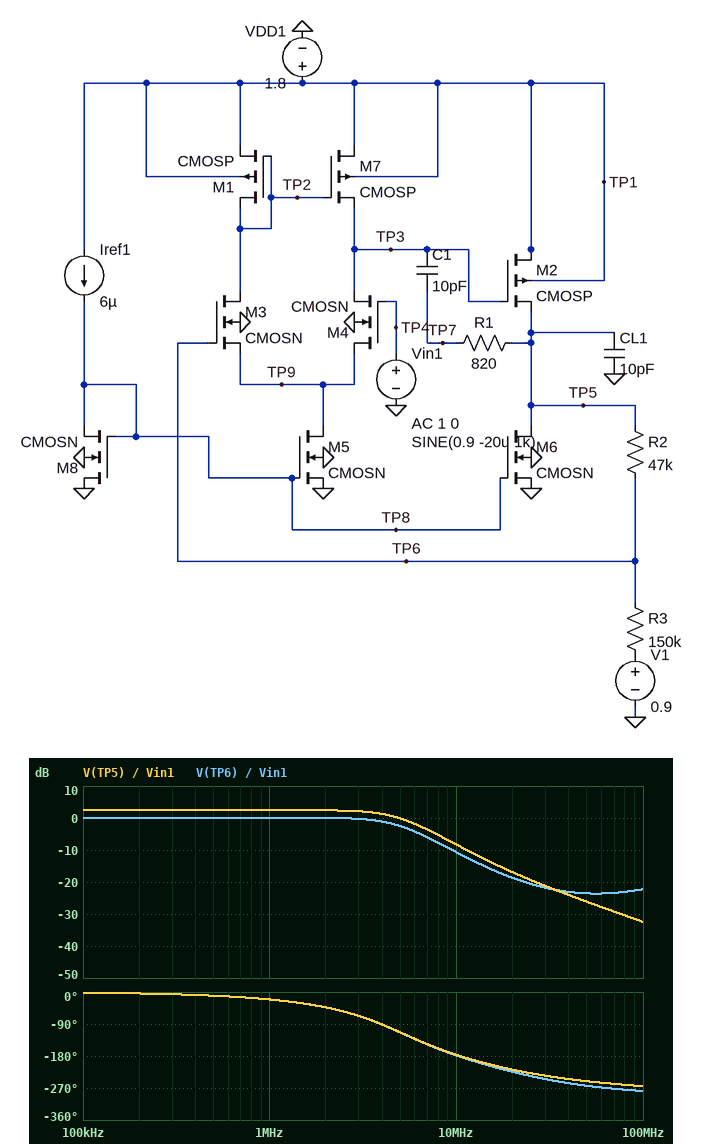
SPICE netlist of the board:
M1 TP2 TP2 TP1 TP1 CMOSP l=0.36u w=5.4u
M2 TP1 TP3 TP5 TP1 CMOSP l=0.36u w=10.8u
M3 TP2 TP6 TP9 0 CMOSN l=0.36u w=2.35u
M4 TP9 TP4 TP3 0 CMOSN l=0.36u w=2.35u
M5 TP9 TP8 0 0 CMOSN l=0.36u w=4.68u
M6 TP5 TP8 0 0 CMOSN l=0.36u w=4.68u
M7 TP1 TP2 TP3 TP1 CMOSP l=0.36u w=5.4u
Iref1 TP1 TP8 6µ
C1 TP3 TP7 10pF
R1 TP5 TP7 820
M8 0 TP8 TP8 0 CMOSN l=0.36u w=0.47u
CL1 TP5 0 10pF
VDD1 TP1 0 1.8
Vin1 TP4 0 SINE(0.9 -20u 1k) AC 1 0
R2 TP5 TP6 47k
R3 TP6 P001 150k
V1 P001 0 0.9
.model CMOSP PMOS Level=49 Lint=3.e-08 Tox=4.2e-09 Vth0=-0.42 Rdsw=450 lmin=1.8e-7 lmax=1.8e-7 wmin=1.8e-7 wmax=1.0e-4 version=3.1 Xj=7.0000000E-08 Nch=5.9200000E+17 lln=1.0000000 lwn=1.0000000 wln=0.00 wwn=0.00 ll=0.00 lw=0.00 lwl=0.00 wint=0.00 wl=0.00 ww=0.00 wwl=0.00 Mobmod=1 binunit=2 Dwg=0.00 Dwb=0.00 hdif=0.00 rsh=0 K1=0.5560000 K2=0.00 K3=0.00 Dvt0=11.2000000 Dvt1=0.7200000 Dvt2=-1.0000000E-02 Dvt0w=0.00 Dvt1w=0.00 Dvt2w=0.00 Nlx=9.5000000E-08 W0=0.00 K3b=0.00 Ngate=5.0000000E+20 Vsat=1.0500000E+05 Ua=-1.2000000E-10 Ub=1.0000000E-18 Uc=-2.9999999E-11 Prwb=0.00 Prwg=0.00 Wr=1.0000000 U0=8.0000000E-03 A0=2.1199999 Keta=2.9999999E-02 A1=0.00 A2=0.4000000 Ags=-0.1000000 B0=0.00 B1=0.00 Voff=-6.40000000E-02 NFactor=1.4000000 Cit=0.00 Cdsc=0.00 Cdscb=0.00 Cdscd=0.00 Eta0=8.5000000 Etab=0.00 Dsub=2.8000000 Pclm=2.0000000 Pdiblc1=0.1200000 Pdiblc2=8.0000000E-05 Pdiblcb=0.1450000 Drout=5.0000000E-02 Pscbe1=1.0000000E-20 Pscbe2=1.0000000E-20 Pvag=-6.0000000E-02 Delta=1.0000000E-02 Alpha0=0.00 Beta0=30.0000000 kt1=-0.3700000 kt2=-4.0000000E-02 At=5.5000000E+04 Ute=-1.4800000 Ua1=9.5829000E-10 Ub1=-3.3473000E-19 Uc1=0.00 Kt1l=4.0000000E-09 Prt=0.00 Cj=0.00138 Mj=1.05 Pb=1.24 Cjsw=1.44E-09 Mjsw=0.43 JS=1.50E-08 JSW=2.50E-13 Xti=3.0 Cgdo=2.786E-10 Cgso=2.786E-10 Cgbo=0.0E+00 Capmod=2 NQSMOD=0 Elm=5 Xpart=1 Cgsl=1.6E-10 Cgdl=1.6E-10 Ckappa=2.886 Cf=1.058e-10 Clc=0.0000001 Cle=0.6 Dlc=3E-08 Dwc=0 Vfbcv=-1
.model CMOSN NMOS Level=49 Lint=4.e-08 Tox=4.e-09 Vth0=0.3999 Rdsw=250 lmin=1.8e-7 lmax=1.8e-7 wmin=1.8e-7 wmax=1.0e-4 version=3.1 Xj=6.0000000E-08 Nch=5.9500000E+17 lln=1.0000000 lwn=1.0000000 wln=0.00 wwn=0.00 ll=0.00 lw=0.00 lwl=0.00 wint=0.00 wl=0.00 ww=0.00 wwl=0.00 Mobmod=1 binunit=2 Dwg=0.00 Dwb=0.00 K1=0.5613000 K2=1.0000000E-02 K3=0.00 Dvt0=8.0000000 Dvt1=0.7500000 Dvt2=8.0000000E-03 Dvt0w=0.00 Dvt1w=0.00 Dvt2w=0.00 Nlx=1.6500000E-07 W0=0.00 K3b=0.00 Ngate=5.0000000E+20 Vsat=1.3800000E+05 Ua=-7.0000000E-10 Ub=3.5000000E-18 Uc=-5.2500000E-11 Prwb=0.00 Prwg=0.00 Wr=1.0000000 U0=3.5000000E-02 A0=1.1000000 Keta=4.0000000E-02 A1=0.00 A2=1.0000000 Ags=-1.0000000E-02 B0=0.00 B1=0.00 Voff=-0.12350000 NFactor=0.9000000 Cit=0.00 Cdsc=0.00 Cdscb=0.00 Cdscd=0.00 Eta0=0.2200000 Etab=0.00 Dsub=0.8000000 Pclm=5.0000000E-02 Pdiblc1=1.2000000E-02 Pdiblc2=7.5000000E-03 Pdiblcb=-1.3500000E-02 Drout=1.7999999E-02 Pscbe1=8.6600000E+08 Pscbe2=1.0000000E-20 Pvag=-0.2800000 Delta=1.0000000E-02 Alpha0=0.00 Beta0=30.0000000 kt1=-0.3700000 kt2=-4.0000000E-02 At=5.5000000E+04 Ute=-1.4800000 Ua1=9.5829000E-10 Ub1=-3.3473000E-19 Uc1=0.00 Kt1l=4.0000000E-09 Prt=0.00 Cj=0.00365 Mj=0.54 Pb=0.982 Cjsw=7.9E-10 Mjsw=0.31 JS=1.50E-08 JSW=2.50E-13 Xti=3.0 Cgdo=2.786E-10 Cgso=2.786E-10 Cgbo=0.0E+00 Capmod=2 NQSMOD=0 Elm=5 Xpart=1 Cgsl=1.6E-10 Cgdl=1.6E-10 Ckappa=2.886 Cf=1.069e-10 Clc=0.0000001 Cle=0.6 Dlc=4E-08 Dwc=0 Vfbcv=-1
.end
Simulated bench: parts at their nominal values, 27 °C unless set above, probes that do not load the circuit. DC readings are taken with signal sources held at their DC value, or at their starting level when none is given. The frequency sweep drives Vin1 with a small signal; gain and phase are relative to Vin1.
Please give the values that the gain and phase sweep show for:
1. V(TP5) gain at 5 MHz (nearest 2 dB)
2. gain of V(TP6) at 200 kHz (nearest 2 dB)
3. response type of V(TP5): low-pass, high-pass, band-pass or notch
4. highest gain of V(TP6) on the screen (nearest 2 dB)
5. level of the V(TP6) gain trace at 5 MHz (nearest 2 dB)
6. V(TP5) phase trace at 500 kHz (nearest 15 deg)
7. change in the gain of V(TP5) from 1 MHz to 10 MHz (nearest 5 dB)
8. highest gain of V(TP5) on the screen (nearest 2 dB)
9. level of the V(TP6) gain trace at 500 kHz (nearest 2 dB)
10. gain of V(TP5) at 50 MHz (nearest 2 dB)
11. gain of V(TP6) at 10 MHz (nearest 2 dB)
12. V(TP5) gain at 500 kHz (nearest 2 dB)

0 dB
0 dB
low-pass
0 dB
-2 dB
-15 deg
-10 dB
2 dB
0 dB
-26 dB
-10 dB
2 dB
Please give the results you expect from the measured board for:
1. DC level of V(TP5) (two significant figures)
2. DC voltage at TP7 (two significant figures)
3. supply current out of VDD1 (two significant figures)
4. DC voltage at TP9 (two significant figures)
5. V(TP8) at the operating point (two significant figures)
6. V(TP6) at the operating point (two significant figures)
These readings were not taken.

900 mV
900 mV
120 µA
180 mV
680 mV
900 mV
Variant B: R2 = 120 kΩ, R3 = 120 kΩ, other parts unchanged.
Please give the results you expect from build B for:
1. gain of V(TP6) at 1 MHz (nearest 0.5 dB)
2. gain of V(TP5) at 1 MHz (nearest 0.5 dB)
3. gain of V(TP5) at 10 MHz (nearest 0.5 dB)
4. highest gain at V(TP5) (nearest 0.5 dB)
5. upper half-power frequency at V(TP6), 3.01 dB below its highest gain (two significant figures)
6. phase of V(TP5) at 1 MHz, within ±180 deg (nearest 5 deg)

-0.5 dB
5.5 dB
-9.0 dB
6.0 dB
2.9 MHz
-30 deg
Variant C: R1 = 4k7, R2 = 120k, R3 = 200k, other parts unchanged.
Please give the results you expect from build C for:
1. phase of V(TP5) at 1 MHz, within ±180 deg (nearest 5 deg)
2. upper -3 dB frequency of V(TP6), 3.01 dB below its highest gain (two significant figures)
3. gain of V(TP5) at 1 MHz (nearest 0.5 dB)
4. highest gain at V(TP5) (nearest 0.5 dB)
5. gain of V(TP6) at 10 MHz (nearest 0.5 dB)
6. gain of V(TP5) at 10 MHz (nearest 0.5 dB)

-25 deg
2.1 MHz
3.0 dB
4.0 dB
-12.0 dB
-7.5 dB
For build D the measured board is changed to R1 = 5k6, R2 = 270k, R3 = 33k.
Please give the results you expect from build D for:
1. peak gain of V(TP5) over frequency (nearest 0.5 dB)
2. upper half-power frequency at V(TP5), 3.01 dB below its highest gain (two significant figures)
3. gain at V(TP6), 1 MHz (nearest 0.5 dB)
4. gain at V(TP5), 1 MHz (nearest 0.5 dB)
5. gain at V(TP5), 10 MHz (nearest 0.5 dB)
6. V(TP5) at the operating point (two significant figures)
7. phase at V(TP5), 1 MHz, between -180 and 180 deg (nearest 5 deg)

19.0 dB
390 kHz
-9.0 dB
10.5 dB
-5.0 dB
890 mV
-65 deg
